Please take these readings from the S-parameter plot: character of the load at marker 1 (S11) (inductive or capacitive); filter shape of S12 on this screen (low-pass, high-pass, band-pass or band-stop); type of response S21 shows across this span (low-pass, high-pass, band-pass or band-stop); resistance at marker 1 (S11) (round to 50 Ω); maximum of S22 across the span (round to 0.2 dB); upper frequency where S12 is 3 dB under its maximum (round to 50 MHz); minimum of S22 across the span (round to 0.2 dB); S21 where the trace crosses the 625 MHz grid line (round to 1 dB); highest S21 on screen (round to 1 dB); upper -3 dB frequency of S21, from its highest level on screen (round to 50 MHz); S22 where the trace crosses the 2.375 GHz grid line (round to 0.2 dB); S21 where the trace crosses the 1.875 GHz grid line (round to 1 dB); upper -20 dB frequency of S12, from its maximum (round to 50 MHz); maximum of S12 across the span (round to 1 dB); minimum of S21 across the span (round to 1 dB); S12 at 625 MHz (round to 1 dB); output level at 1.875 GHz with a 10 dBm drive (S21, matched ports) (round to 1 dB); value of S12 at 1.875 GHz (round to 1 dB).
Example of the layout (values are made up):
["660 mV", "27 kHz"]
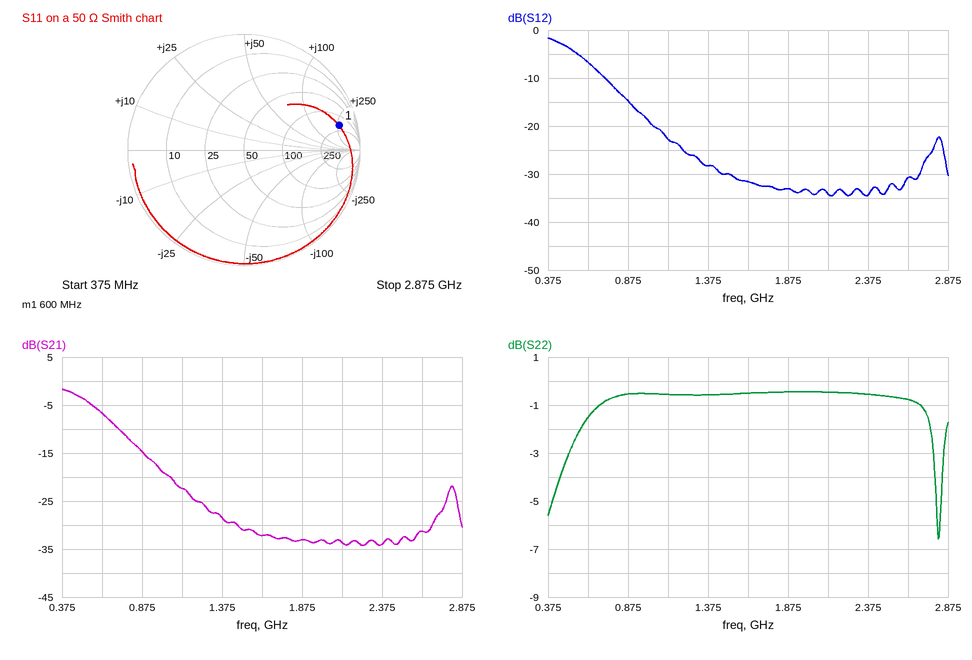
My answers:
["inductive", "low-pass", "low-pass", "200 Ω", "-0.4 dB", "550 MHz", "-6.6 dB", "-7 dB", "-2 dB", "550 MHz", "-0.6 dB", "-33 dB", "1.10 GHz", "-2 dB", "-34 dB", "-7 dB", "-23 dBm", "-33 dB"]
